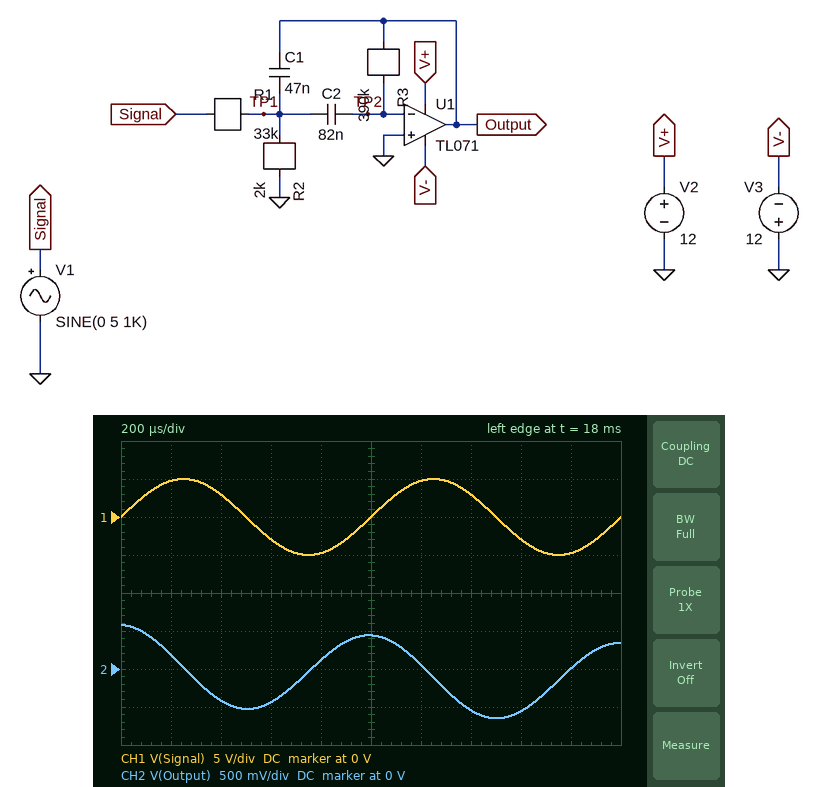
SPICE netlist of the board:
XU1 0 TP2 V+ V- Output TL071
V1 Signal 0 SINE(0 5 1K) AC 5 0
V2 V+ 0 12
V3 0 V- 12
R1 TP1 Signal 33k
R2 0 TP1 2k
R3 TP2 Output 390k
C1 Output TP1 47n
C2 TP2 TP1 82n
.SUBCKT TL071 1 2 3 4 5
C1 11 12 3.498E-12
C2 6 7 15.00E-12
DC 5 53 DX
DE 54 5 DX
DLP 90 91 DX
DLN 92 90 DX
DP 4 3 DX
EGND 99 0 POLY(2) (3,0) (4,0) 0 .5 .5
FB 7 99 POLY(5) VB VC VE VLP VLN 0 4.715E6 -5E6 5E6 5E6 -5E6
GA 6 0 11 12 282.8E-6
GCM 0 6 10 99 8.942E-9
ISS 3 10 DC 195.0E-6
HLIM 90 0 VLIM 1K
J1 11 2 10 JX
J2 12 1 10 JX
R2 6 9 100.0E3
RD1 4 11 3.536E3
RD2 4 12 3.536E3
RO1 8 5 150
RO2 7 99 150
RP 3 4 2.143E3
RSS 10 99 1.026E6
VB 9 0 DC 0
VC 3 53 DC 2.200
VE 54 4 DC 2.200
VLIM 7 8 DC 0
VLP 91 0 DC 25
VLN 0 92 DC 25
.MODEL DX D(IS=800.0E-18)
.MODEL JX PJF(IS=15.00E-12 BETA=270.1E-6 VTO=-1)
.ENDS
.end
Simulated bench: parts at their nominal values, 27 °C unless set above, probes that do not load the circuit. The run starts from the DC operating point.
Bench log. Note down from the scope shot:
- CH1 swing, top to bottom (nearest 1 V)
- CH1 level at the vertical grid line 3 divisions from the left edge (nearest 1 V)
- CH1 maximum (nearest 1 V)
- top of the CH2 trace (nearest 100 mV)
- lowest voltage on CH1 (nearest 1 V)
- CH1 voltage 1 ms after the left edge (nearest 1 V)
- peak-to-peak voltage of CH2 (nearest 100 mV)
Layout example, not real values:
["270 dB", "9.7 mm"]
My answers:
["10 V", "-3 V", "5 V", "600 mV", "-5 V", "0 V", "1.2 V"]
